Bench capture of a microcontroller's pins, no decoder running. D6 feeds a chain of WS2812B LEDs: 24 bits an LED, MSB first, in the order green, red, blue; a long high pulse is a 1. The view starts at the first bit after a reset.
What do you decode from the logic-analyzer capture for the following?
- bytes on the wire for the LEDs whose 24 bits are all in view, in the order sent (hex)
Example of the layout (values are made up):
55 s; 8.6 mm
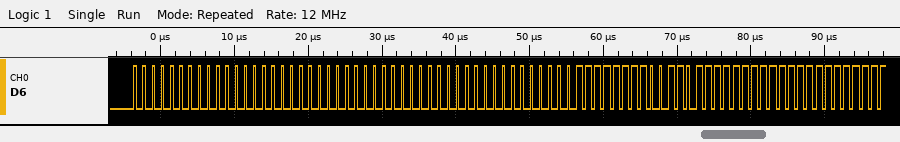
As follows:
00 00 00 00 00 00 FF 37 FF
